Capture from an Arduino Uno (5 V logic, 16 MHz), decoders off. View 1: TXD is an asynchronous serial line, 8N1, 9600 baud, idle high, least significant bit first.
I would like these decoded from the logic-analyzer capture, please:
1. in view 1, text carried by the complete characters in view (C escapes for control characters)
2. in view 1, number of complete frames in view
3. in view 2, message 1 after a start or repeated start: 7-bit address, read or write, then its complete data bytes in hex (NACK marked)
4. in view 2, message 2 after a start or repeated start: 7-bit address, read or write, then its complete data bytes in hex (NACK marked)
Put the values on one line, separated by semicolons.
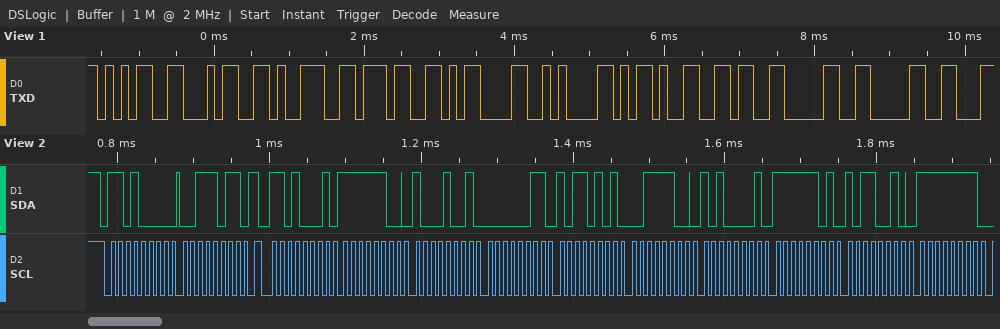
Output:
"5497\r\n-600"; 10; 0x68 write: 3B; 0x68 read: FC 89 03 B5 3C A1 FD B2 FF
